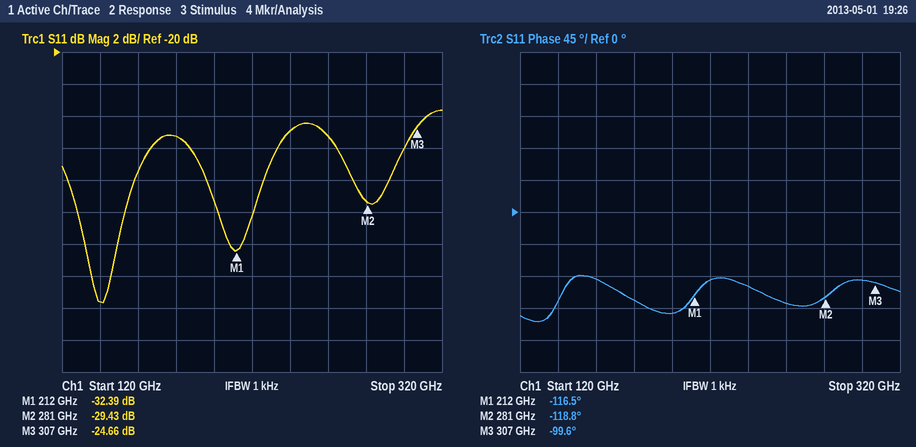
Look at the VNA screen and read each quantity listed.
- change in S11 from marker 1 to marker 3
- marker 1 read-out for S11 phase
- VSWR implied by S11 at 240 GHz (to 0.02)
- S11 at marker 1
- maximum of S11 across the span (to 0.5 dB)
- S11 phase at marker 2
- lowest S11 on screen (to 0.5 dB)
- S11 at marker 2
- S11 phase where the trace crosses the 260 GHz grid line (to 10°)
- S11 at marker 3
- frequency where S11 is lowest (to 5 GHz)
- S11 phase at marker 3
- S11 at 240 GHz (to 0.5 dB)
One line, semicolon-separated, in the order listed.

7.73 dB; -116.5°; 1.12; -32.39 dB; -23.5 dB; -118.8°; -35.5 dB; -29.43 dB; -130°; -24.66 dB; 140 GHz; -99.6°; -25.0 dB
